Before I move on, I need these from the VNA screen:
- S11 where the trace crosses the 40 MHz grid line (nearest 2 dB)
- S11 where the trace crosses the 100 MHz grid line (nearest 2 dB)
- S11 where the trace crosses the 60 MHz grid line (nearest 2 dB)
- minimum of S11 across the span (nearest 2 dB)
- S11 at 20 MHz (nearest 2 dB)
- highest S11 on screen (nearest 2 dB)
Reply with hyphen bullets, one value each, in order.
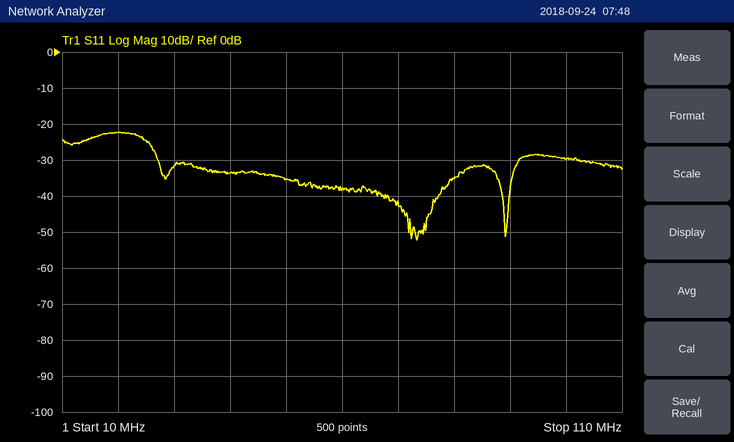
- -34 dB
- -30 dB
- -38 dB
- -52 dB
- -22 dB
- -22 dB
